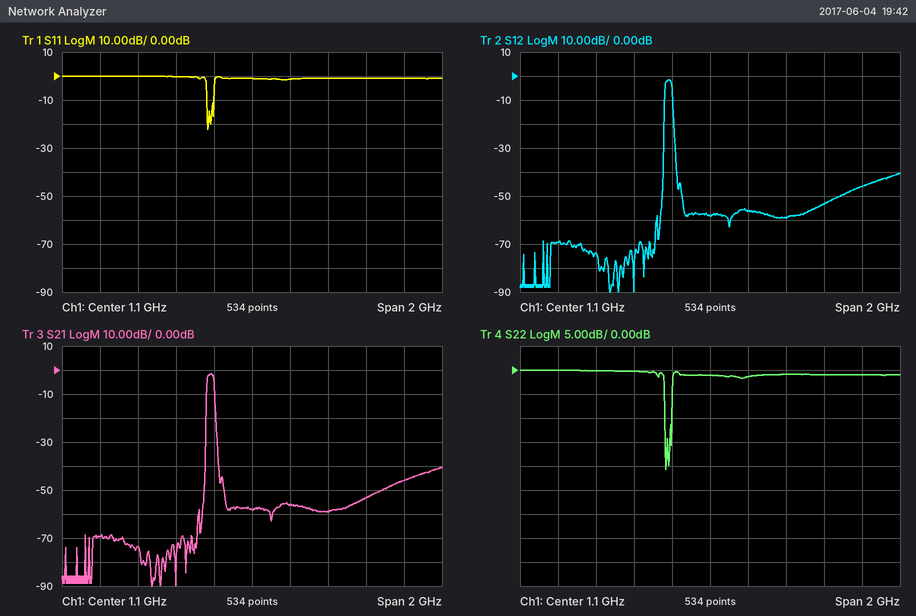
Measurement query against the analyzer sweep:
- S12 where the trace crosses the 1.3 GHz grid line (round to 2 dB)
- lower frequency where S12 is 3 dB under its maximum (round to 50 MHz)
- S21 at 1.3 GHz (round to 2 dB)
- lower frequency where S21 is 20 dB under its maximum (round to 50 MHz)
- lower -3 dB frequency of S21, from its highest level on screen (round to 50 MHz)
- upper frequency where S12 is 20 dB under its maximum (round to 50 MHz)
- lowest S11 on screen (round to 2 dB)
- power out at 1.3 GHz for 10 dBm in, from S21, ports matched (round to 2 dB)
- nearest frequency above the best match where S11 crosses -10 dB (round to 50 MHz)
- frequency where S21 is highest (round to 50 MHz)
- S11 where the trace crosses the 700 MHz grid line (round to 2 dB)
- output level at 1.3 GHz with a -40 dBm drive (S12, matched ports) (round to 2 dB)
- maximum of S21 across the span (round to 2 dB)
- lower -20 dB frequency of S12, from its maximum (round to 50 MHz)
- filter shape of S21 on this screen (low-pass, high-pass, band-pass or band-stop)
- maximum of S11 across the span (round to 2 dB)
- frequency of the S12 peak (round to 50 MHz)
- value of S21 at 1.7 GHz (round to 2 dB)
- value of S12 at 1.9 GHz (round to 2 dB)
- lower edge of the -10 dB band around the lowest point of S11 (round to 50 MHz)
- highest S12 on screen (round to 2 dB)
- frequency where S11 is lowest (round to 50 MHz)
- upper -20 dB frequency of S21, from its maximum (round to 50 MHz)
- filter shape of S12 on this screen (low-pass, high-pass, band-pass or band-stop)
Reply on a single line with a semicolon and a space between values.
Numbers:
-56 dB; 850 MHz; -56 dB; 850 MHz; 850 MHz; 900 MHz; -22 dB; -46 dBm; 900 MHz; 900 MHz; 0 dB; -96 dBm; -2 dB; 850 MHz; band-pass; 0 dB; 900 MHz; -54 dB; -46 dB; 850 MHz; -2 dB; 850 MHz; 900 MHz; band-pass
